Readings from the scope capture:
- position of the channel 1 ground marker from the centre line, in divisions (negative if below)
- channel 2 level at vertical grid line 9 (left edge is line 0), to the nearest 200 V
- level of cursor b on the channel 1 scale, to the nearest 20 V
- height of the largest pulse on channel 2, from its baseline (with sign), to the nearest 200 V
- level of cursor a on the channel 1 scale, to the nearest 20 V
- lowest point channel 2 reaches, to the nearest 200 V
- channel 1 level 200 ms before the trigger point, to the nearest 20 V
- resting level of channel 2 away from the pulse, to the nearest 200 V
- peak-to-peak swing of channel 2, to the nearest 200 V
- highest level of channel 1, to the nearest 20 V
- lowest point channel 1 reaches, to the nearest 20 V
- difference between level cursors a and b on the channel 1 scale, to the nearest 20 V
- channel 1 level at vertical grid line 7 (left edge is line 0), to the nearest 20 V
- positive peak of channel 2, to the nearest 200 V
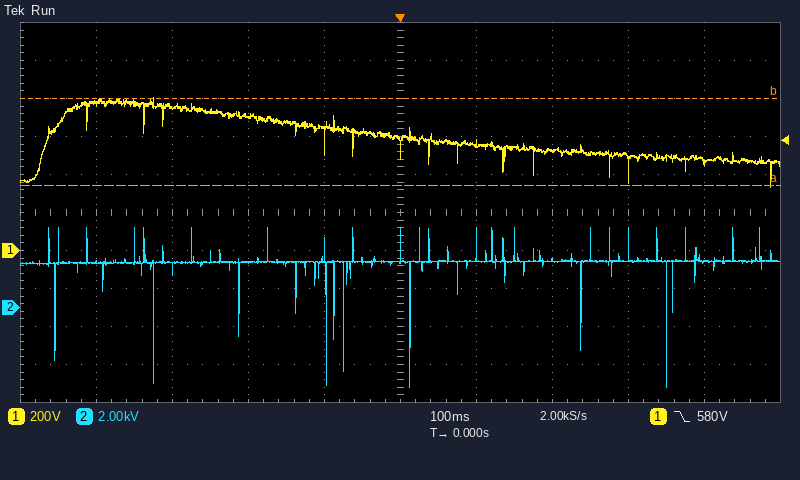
-1.0 div
2.4 kV
800 V
-6.6 kV
340 V
-4.2 kV
700 V
2.4 kV
8.4 kV
800 V
340 V
460 V
520 V
4.2 kV
